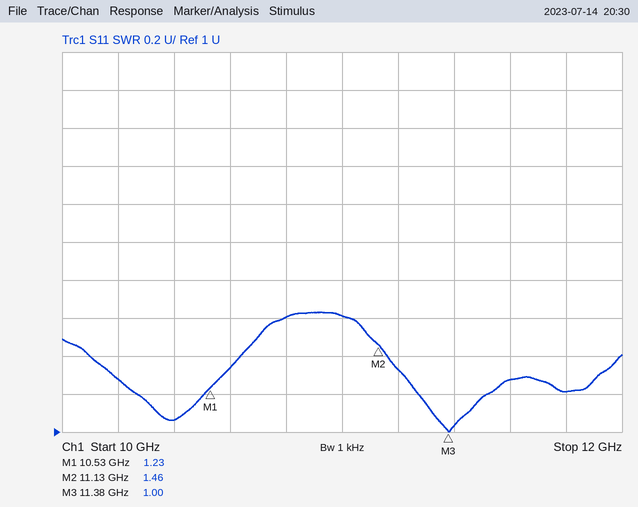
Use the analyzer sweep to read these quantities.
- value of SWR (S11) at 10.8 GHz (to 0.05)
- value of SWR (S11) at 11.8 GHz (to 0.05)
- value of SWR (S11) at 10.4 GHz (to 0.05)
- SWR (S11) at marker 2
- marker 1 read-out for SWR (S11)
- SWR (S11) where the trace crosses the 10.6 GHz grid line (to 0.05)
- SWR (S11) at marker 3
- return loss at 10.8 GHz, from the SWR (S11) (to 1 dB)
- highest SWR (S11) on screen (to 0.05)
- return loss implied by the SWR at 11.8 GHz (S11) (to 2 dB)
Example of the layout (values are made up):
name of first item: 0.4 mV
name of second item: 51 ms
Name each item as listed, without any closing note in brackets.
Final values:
value of SWR (S11) at 10.8 GHz: 1.60
value of SWR (S11) at 11.8 GHz: 1.20
value of SWR (S11) at 10.4 GHz: 1.05
SWR (S11) at marker 2: 1.46
marker 1 read-out for SWR: 1.23
SWR (S11) where the trace crosses the 10.6 GHz grid line: 1.35
SWR (S11) at marker 3: 1.00
return loss at 10.8 GHz, from the SWR (S11): 13 dB
highest SWR (S11) on screen: 1.65
return loss implied by the SWR at 11.8 GHz (S11): 20 dB
